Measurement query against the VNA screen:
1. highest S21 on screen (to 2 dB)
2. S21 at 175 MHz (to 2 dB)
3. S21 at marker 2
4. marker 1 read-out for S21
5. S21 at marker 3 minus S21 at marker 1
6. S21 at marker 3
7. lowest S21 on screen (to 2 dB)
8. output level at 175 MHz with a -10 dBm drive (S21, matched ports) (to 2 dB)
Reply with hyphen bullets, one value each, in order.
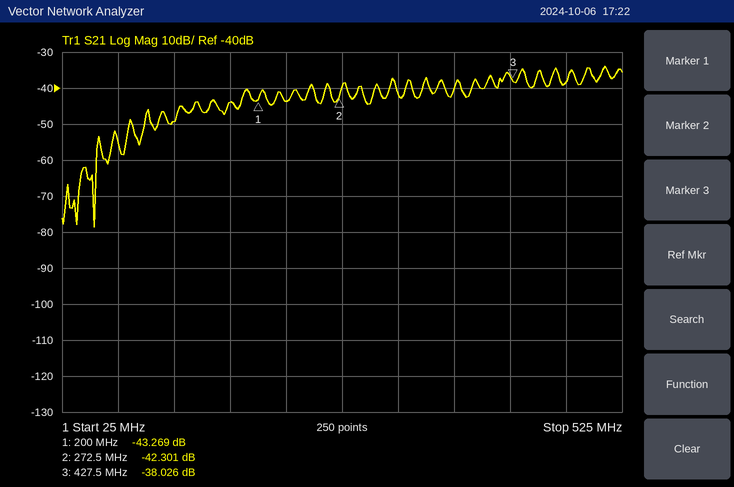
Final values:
- -34 dB
- -44 dB
- -42.301 dB
- -43.269 dB
- 5.243 dB
- -38.026 dB
- -78 dB
- -54 dBm
